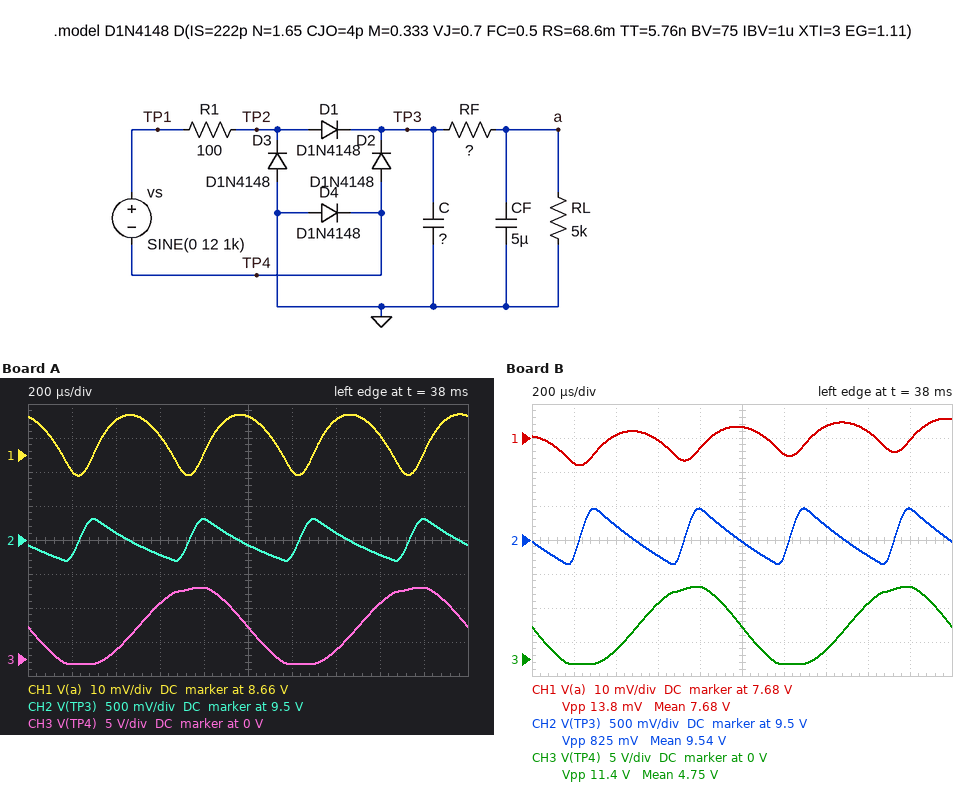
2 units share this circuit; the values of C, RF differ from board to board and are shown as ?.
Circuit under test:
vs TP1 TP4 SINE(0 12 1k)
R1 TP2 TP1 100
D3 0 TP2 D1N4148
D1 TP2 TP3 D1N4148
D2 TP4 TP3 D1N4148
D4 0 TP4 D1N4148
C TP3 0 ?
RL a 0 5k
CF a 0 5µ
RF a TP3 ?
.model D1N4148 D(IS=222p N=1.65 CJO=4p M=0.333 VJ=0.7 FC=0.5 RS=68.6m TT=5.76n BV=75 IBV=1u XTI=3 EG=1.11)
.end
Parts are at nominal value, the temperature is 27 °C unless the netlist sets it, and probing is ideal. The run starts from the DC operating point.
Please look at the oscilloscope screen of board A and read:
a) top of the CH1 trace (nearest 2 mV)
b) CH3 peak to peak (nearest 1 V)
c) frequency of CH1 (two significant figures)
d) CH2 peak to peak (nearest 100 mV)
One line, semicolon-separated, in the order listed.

8.672 V; 11 V; 2.0 kHz; 600 mV
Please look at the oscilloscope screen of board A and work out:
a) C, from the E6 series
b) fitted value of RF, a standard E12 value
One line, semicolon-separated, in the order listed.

1 µF; 470 Ω
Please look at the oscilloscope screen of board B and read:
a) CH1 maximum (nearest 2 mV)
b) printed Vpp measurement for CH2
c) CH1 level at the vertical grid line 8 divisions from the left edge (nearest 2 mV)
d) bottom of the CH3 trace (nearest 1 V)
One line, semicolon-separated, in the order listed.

7.686 V; 825 mV; 7.682 V; -1 V
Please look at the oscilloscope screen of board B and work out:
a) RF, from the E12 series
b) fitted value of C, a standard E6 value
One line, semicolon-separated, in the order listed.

1.2 kΩ; 680 nF
